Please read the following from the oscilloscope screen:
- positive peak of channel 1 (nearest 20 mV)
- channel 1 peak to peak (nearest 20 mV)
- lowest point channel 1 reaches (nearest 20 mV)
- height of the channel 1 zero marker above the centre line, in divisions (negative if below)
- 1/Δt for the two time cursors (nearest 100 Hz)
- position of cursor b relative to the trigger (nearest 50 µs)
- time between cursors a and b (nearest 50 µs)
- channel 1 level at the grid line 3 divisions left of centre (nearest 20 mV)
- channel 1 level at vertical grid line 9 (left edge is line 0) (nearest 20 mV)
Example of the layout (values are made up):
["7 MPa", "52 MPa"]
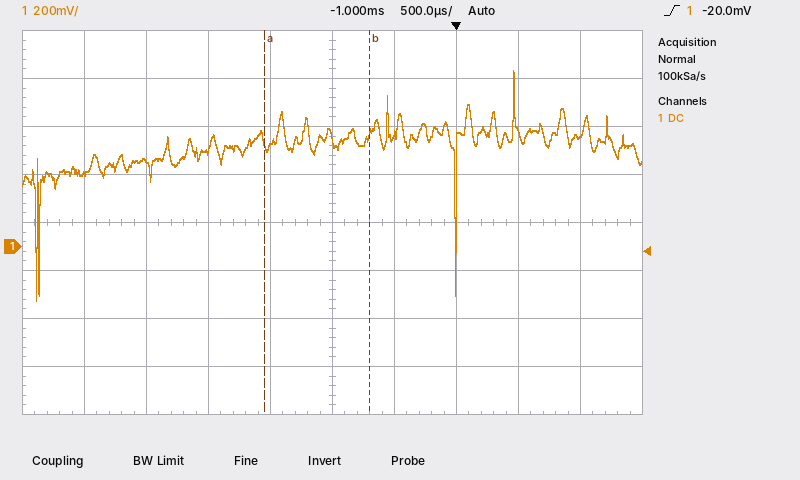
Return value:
["740 mV", "960 mV", "-220 mV", "-0.5 div", "1.2 kHz", "-700 µs", "850 µs", "360 mV", "460 mV"]
